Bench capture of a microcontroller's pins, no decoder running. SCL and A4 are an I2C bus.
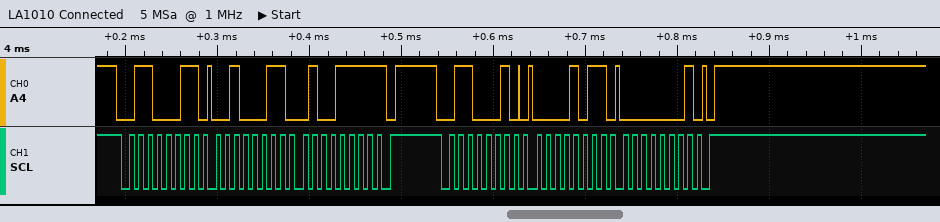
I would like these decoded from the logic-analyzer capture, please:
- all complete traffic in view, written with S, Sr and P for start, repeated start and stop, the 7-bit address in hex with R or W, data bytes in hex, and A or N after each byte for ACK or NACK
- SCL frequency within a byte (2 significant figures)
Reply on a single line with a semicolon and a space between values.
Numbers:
S 31R A 23 A 4F N P S 31W A 0B A 01 A P; 100 kHz
